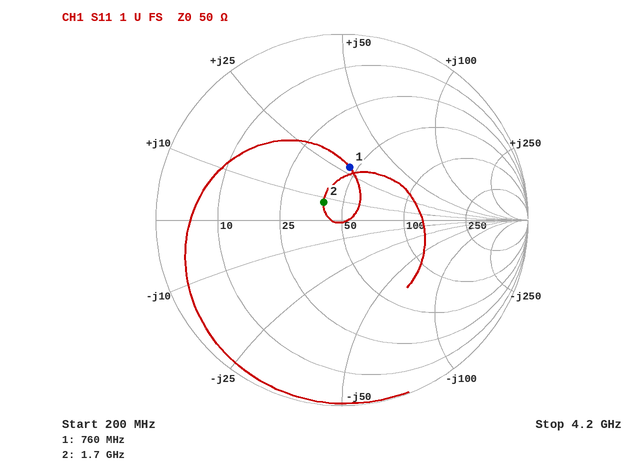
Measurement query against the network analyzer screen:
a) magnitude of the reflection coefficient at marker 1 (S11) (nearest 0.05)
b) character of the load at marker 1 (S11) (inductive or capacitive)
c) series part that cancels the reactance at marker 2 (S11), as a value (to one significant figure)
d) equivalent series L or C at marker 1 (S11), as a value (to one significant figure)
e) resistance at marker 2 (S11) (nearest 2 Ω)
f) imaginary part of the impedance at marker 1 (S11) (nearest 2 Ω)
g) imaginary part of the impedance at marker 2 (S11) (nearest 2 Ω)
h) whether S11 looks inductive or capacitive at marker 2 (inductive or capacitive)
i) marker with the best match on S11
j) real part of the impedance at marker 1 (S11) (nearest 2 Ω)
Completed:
0.30
inductive
10 pF
6 nH
40 Ω
+28 Ω
+8 Ω
inductive
marker 2
46 Ω
